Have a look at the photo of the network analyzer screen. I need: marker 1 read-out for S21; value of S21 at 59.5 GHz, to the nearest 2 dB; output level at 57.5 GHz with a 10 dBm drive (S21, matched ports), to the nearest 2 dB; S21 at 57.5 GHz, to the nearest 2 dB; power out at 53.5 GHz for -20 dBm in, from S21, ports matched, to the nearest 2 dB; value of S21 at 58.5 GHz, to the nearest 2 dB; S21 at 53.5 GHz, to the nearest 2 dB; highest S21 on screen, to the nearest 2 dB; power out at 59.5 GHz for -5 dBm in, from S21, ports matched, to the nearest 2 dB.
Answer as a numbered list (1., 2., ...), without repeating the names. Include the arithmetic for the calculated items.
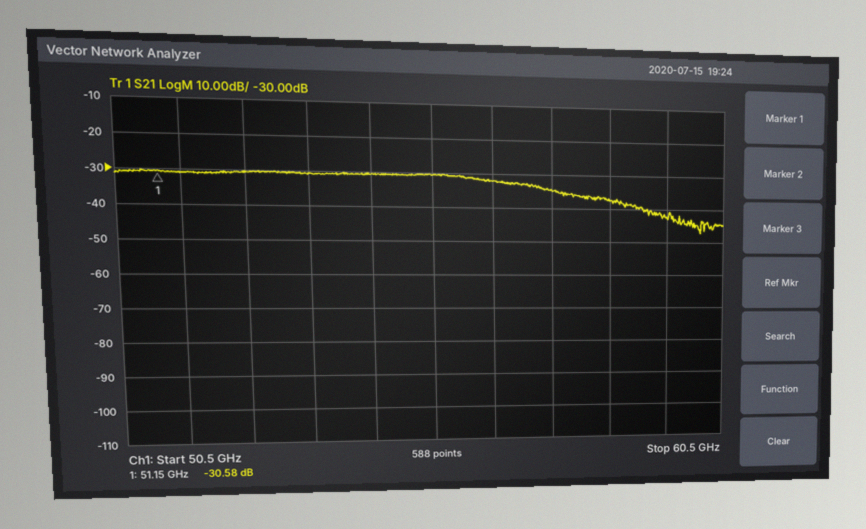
1. -30.58 dB
2. -42 dB
3. 10 dBm + (-34 dB) = -24 dBm
4. -34 dB
5. -20 dBm + (-30 dB) = -50 dBm
6. -38 dB
7. -30 dB
8. -30 dB
9. -5 dBm + (-42 dB) = -48 dBm
